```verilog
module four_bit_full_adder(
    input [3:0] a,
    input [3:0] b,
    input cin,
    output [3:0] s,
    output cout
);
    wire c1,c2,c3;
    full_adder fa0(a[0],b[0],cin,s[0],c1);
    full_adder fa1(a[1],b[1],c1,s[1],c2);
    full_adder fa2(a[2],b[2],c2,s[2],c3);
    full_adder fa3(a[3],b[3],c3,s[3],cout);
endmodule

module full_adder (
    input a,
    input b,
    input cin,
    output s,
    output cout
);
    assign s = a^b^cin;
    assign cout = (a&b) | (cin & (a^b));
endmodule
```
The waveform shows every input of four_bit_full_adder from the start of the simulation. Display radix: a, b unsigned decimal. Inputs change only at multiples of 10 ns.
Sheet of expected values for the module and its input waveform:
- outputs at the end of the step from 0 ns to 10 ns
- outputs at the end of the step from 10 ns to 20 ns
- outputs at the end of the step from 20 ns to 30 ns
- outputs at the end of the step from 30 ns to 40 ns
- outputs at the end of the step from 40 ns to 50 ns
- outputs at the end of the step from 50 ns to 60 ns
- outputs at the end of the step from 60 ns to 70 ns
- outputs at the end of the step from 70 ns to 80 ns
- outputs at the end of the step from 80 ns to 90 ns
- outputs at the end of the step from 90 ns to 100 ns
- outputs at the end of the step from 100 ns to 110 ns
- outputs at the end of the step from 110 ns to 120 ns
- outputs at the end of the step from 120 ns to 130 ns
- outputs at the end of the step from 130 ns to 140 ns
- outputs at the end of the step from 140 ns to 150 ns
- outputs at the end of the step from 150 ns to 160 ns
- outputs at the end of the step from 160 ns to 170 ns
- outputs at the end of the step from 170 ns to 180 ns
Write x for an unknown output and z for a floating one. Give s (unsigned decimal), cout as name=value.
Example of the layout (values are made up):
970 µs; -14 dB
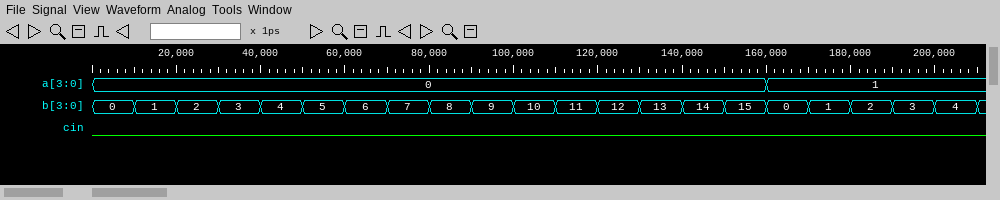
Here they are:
s=0, cout=0; s=1, cout=0; s=2, cout=0; s=3, cout=0; s=4, cout=0; s=5, cout=0; s=6, cout=0; s=7, cout=0; s=8, cout=0; s=9, cout=0; s=10, cout=0; s=11, cout=0; s=12, cout=0; s=13, cout=0; s=14, cout=0; s=15, cout=0; s=1, cout=0; s=2, cout=0
